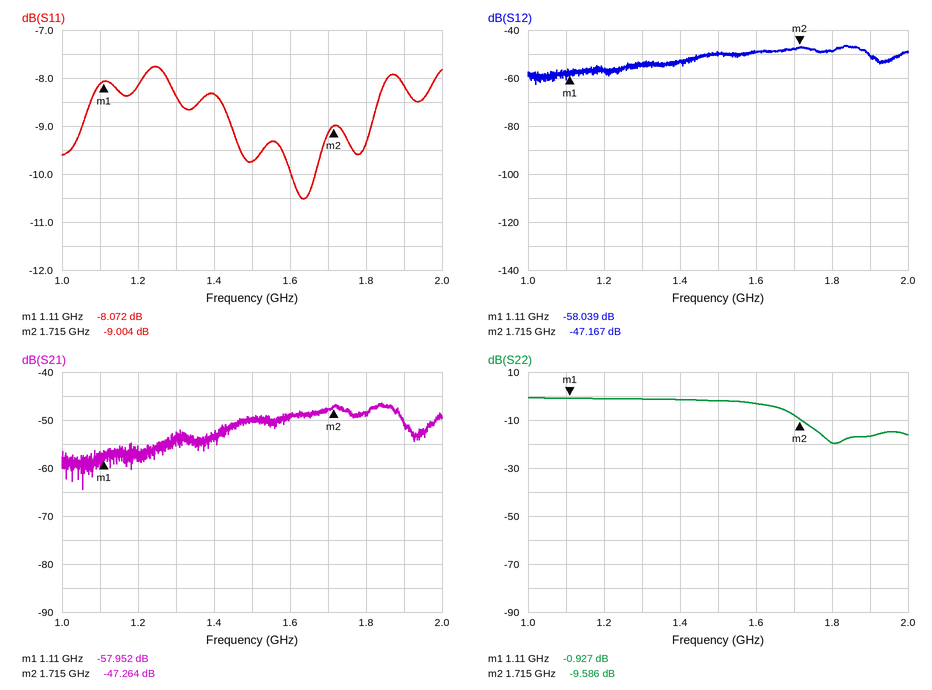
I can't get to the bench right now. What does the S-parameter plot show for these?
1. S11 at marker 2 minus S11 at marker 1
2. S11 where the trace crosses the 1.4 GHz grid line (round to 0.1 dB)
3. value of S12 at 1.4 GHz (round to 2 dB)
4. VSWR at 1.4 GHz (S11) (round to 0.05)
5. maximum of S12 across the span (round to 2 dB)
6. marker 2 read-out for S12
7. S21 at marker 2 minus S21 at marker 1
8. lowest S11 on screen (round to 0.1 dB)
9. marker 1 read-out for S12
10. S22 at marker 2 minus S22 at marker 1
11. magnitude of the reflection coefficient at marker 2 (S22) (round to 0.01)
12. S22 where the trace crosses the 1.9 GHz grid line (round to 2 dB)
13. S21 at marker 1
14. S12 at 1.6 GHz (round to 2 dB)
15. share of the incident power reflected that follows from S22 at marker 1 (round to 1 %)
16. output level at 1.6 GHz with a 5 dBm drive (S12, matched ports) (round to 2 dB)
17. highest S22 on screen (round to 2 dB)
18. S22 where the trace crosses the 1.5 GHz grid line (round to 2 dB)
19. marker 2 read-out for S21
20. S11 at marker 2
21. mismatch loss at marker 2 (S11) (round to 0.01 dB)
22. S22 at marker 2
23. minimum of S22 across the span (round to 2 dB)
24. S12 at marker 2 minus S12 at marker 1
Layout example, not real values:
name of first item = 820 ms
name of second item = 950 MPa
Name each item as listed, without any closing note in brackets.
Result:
S11 at marker 2 minus S11 at marker 1 = -0.932 dB
S11 where the trace crosses the 1.4 GHz grid line = -8.3 dB
value of S12 at 1.4 GHz = -54 dB
VSWR at 1.4 GHz (S11) = 2.25
maximum of S12 across the span = -46 dB
marker 2 read-out for S12 = -47.167 dB
S21 at marker 2 minus S21 at marker 1 = 10.688 dB
lowest S11 on screen = -10.5 dB
marker 1 read-out for S12 = -58.039 dB
S22 at marker 2 minus S22 at marker 1 = -8.659 dB
magnitude of the reflection coefficient at marker 2 (S22) = 0.33
S22 where the trace crosses the 1.9 GHz grid line = -16 dB
S21 at marker 1 = -57.952 dB
S12 at 1.6 GHz = -50 dB
share of the incident power reflected that follows from S22 at marker 1 = 81 %
output level at 1.6 GHz with a 5 dBm drive (S12, matched ports) = -44 dBm
highest S22 on screen = 0 dB
S22 where the trace crosses the 1.5 GHz grid line = -2 dB
marker 2 read-out for S21 = -47.264 dB
S11 at marker 2 = -9.004 dB
mismatch loss at marker 2 (S11) = 0.58 dB
S22 at marker 2 = -9.586 dB
minimum of S22 across the span = -20 dB
S12 at marker 2 minus S12 at marker 1 = 10.872 dB
